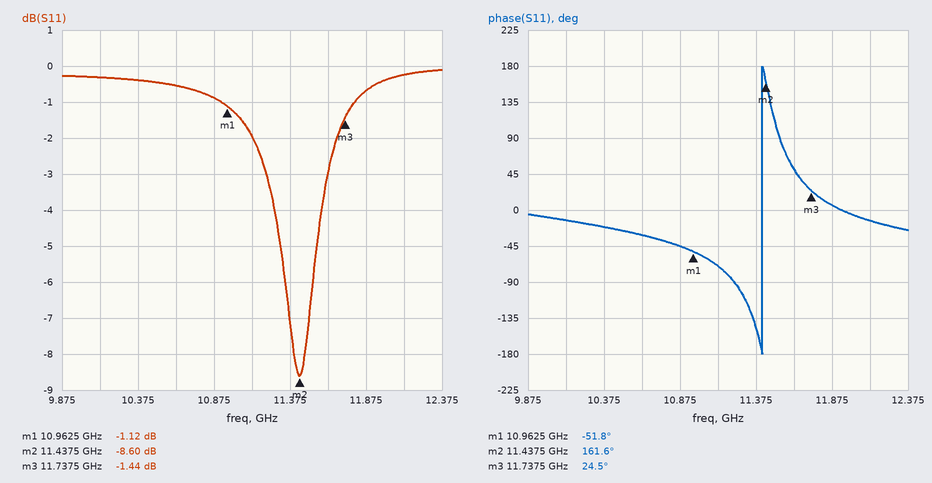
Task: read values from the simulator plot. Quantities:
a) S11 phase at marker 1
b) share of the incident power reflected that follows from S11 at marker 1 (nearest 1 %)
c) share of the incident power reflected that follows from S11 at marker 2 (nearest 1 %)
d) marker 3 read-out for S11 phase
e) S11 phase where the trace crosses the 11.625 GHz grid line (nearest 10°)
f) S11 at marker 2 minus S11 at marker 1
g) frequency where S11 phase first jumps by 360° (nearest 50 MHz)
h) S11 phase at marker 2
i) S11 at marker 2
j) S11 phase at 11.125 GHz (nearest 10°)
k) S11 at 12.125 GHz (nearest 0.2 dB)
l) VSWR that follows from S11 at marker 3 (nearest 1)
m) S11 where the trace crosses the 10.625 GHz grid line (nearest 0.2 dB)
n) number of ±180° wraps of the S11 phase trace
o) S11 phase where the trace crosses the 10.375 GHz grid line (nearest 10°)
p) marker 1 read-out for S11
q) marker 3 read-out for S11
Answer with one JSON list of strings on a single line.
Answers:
["-51.8°", "77 %", "14 %", "24.5°", "50°", "-7.48 dB", "11.40 GHz", "161.6°", "-8.60 dB", "-70°", "-0.2 dB", "12", "-0.6 dB", "1", "-20°", "-1.12 dB", "-1.44 dB"]
